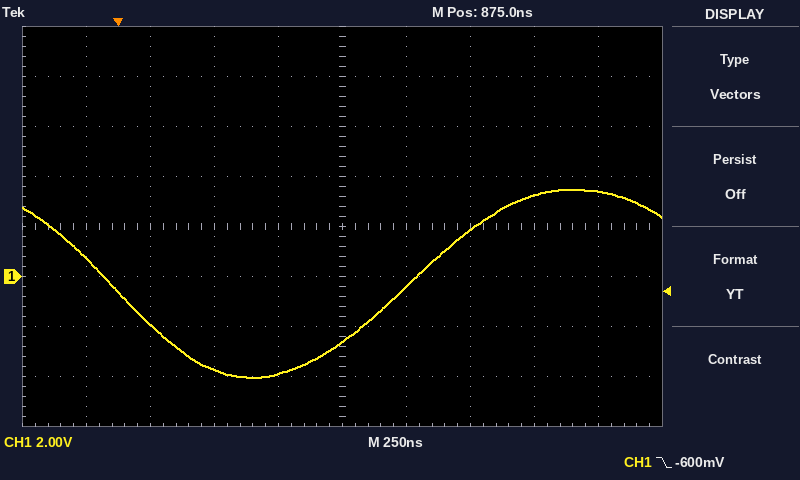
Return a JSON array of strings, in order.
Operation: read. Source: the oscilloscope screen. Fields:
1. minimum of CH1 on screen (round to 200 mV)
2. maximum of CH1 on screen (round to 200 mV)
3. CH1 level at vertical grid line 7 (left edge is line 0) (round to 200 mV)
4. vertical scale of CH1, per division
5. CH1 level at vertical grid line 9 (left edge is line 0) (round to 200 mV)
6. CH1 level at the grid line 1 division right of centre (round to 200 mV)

["-4.0 V", "3.4 V", "1.8 V", "2 V", "3.4 V", "-400 mV"]
